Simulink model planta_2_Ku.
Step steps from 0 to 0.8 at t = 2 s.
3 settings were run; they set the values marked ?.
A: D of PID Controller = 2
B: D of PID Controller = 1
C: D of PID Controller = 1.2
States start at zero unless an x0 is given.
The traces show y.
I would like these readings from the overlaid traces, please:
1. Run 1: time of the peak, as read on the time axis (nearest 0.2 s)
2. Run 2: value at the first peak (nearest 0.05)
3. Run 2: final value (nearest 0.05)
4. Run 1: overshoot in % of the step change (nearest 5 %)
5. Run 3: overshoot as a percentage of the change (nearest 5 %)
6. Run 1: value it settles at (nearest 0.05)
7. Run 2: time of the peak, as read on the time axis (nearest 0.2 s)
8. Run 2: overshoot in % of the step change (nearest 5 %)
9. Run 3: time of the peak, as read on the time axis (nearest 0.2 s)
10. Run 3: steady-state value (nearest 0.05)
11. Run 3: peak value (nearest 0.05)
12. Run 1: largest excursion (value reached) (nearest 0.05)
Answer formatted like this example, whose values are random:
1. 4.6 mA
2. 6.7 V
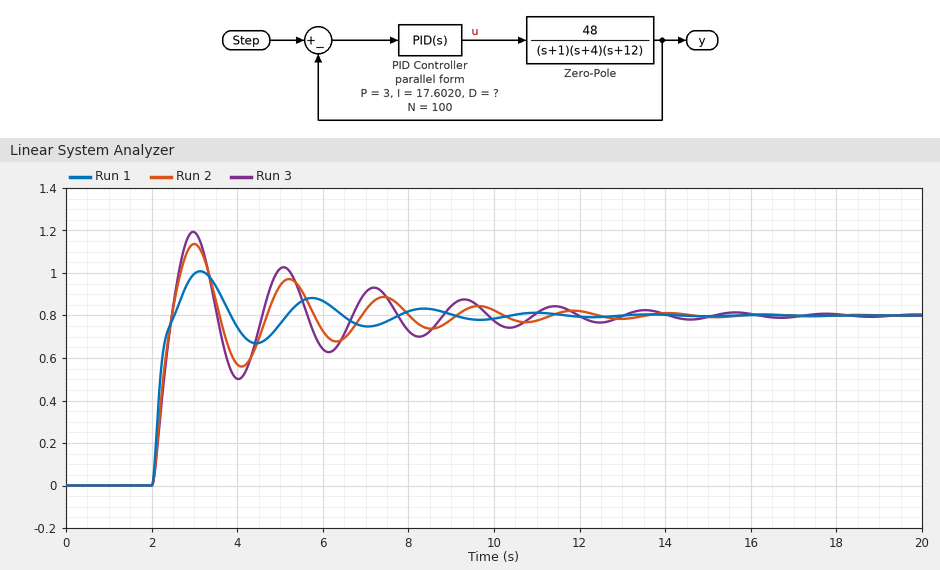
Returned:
1. 3.2 s
2. 1.15
3. 0.80
4. 25 %
5. 50 %
6. 0.80
7. 3.0 s
8. 40 %
9. 3.0 s
10. 0.80
11. 1.20
12. 1.00
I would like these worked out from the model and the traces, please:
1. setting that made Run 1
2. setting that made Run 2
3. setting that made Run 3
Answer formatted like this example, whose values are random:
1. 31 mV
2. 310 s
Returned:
1. A
2. C
3. B
